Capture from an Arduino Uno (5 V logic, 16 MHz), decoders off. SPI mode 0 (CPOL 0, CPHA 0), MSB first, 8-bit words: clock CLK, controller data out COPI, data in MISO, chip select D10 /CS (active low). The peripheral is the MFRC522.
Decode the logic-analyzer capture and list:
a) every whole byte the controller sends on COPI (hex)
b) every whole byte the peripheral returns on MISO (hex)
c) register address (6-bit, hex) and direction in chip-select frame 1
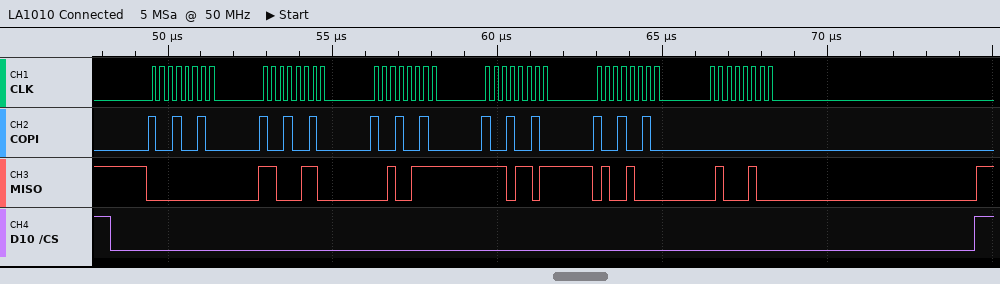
92 92 92 92 92 00
00 C6 27 ED 48 44
0x09 read
